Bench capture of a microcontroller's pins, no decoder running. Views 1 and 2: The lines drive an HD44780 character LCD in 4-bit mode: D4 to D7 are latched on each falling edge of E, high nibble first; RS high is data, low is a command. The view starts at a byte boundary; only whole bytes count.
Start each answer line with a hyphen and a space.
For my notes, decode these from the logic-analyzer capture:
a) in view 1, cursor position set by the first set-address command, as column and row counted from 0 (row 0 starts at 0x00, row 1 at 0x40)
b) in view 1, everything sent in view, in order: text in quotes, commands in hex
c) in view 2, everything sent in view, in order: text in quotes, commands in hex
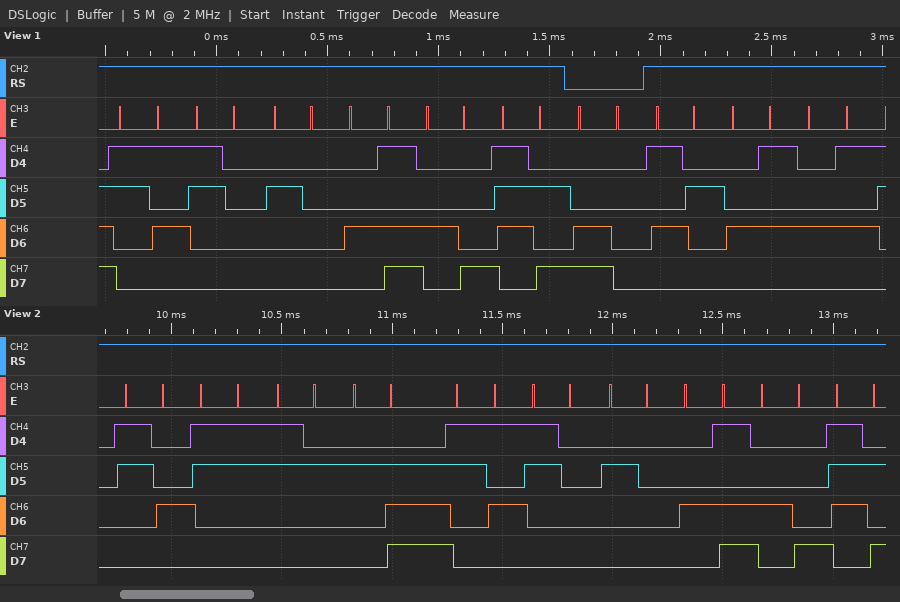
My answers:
- column 0, row 1
- "50 MHz" 0xC0 "REE"
- "432.50 MHz"
